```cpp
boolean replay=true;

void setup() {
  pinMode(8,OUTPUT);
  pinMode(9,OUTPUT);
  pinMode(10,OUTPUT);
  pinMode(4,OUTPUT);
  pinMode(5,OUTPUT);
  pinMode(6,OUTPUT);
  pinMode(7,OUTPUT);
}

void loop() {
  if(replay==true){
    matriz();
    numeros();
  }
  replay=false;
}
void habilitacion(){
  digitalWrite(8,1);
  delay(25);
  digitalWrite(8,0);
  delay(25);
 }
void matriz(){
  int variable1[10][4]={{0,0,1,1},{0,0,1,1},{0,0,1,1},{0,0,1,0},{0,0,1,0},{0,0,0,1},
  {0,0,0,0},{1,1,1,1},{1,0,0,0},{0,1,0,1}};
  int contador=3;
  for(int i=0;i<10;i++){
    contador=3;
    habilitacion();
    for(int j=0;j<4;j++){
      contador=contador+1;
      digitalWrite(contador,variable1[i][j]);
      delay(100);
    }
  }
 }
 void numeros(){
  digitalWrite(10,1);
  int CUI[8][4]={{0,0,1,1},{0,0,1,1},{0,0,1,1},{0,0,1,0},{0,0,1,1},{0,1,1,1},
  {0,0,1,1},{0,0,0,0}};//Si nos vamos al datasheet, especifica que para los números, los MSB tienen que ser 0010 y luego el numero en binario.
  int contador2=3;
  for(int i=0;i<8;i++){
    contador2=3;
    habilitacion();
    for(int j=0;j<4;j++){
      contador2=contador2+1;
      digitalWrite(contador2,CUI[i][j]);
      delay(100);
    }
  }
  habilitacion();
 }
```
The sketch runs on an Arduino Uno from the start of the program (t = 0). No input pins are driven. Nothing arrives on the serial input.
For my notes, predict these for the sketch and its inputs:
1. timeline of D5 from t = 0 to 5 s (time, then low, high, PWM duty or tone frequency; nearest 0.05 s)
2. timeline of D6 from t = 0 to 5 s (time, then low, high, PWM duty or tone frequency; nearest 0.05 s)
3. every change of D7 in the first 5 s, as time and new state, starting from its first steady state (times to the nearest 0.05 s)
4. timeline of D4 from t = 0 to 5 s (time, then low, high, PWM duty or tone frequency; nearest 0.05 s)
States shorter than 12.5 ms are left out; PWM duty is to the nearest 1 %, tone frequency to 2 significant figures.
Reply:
0 s low; 3.3 s high; 3.75 s low; 4.2 s high; 4.65 s low
0 s low; 0.25 s high; 2.5 s low; 3.4 s high; 3.85 s low; 4.75 s high
0 s low; 0.35 s high; 1.7 s low; 2.6 s high; 3.05 s low; 3.5 s high; 3.95 s low; 4.4 s high
0 s low; 3.2 s high; 4.1 s low
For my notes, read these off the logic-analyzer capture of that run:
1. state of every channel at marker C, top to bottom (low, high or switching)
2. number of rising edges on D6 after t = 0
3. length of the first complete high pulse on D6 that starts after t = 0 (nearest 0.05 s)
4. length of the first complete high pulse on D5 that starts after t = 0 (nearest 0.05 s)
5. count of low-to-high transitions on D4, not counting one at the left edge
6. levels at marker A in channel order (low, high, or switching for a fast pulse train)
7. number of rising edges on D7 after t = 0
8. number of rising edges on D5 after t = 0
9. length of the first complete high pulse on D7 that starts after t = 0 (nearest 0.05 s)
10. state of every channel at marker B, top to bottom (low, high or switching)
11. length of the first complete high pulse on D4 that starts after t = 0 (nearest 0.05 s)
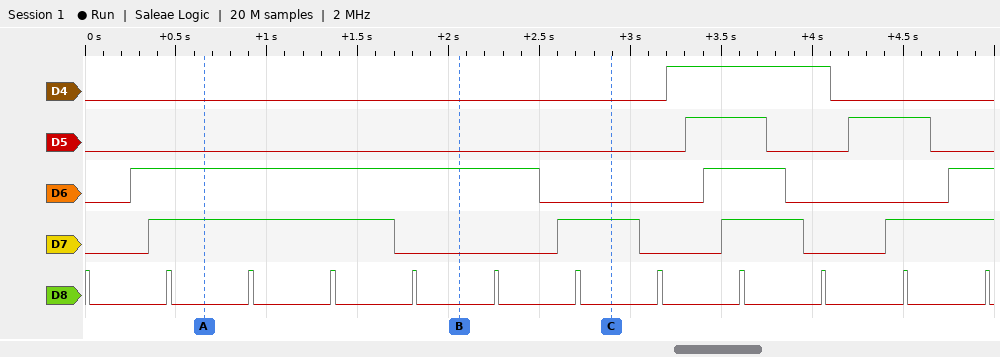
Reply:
D4 low, D5 low, D6 low, D7 high, D8 low
3
2.25 s
0.45 s
1
D4 low, D5 low, D6 high, D7 high, D8 low
4
2
1.35 s
D4 low, D5 low, D6 high, D7 low, D8 low
0.90 s
